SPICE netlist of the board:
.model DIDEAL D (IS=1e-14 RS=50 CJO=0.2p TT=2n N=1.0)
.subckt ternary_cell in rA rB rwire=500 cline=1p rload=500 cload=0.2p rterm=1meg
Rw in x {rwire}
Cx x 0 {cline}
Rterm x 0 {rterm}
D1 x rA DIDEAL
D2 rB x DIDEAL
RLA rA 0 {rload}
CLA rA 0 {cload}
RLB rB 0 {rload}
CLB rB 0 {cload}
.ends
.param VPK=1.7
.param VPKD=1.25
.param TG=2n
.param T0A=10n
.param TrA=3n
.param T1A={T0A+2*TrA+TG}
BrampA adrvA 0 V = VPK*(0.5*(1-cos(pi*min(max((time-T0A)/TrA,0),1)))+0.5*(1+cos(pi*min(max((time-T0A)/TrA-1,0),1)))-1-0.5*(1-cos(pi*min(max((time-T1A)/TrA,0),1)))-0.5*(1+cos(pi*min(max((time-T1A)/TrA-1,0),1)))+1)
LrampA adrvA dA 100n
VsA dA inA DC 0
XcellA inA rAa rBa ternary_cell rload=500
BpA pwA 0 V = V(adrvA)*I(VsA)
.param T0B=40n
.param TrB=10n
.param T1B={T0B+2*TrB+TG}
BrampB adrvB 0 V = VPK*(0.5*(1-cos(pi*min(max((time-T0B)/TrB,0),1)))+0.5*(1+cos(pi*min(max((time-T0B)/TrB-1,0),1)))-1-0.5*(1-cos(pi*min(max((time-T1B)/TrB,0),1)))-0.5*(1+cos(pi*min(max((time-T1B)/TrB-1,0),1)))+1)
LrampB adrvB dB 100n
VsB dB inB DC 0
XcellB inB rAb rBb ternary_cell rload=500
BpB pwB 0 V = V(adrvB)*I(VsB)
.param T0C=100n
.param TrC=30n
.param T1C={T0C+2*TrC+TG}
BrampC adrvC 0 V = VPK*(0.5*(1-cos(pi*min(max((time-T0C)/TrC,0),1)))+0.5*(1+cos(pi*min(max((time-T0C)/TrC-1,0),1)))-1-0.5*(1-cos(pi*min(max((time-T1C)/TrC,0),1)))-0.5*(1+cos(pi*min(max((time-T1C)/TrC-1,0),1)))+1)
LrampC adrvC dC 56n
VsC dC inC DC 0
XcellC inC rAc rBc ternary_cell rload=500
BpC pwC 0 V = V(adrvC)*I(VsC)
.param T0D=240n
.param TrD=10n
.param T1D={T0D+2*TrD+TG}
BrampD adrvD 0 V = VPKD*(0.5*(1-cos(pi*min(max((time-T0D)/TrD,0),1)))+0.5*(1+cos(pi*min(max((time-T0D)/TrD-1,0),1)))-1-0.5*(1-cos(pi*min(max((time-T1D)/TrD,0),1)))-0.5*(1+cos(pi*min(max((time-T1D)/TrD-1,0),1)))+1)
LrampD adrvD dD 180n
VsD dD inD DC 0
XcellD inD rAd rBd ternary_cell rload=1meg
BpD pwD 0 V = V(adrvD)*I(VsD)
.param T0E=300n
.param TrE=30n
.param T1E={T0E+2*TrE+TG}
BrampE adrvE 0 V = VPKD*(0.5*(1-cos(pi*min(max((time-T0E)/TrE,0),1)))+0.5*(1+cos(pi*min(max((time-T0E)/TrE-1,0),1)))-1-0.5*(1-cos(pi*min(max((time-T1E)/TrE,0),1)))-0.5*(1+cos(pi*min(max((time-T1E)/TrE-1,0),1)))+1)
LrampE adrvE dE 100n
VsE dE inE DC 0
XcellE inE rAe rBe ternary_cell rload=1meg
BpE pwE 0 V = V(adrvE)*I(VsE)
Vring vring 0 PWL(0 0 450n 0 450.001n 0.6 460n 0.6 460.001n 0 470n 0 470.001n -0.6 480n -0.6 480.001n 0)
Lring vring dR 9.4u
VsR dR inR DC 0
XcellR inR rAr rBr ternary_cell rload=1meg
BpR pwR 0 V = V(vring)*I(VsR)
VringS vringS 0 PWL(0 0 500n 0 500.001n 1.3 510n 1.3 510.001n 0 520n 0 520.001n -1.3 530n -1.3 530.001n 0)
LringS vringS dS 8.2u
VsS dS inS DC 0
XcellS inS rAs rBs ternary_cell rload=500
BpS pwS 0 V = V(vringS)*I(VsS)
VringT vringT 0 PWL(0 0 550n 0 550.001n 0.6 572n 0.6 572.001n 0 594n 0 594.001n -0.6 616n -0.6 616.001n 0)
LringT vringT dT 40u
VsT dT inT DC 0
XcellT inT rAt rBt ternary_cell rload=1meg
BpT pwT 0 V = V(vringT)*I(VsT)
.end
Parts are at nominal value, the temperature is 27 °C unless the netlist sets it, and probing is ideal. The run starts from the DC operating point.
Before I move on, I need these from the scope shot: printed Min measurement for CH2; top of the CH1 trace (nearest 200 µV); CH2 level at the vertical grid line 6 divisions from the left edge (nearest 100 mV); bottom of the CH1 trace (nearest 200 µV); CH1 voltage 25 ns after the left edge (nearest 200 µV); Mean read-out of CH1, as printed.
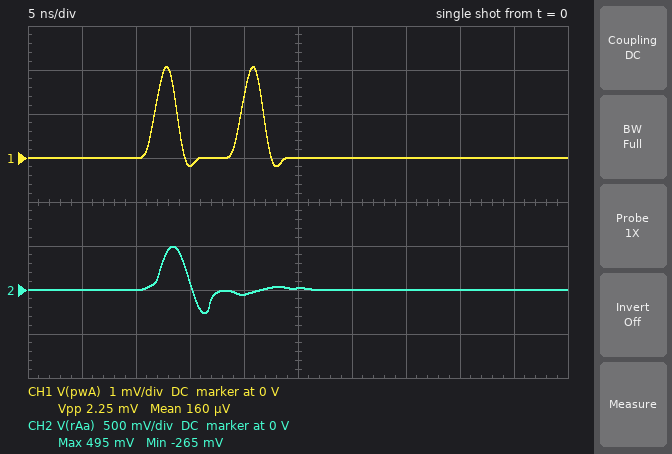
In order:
-265 mV
2.0 mV
0 V
-200 µV
0 V
160 µV
